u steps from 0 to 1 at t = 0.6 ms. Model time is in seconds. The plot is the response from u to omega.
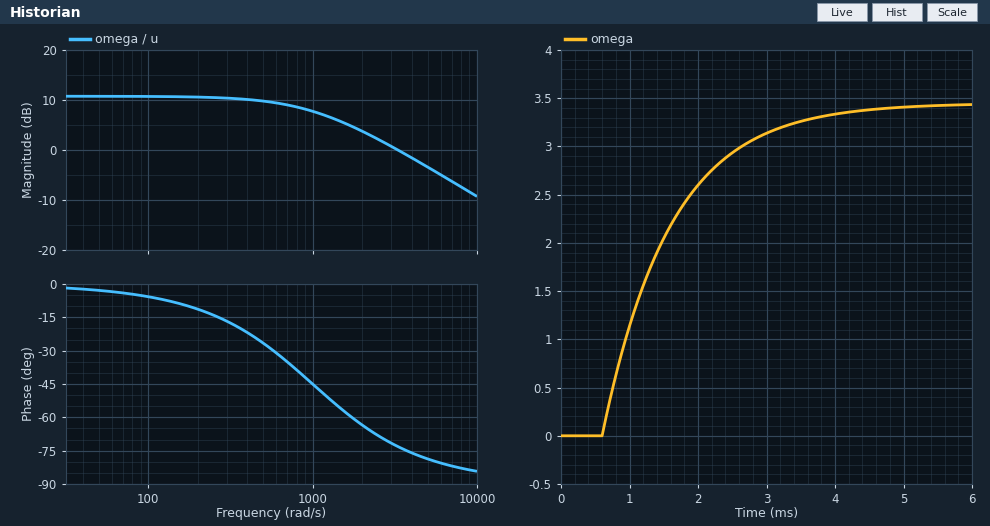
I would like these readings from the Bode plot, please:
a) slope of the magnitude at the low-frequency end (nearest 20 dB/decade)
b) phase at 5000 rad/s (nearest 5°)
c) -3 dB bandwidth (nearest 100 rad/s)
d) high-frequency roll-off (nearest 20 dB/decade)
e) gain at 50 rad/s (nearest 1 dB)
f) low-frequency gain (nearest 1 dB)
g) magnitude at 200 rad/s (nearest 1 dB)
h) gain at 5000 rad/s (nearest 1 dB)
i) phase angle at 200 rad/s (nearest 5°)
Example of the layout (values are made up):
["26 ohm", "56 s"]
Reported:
["0 dB/decade", "-80°", "1000 rad/s", "-20 dB/decade", "11 dB", "11 dB", "11 dB", "-3 dB", "-10°"]
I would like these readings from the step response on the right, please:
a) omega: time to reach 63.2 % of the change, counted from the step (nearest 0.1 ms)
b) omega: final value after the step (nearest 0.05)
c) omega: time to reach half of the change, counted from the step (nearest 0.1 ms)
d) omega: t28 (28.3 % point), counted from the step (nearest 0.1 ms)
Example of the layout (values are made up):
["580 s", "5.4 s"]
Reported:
["1.0 ms", "3.45", "0.7 ms", "0.3 ms"]
